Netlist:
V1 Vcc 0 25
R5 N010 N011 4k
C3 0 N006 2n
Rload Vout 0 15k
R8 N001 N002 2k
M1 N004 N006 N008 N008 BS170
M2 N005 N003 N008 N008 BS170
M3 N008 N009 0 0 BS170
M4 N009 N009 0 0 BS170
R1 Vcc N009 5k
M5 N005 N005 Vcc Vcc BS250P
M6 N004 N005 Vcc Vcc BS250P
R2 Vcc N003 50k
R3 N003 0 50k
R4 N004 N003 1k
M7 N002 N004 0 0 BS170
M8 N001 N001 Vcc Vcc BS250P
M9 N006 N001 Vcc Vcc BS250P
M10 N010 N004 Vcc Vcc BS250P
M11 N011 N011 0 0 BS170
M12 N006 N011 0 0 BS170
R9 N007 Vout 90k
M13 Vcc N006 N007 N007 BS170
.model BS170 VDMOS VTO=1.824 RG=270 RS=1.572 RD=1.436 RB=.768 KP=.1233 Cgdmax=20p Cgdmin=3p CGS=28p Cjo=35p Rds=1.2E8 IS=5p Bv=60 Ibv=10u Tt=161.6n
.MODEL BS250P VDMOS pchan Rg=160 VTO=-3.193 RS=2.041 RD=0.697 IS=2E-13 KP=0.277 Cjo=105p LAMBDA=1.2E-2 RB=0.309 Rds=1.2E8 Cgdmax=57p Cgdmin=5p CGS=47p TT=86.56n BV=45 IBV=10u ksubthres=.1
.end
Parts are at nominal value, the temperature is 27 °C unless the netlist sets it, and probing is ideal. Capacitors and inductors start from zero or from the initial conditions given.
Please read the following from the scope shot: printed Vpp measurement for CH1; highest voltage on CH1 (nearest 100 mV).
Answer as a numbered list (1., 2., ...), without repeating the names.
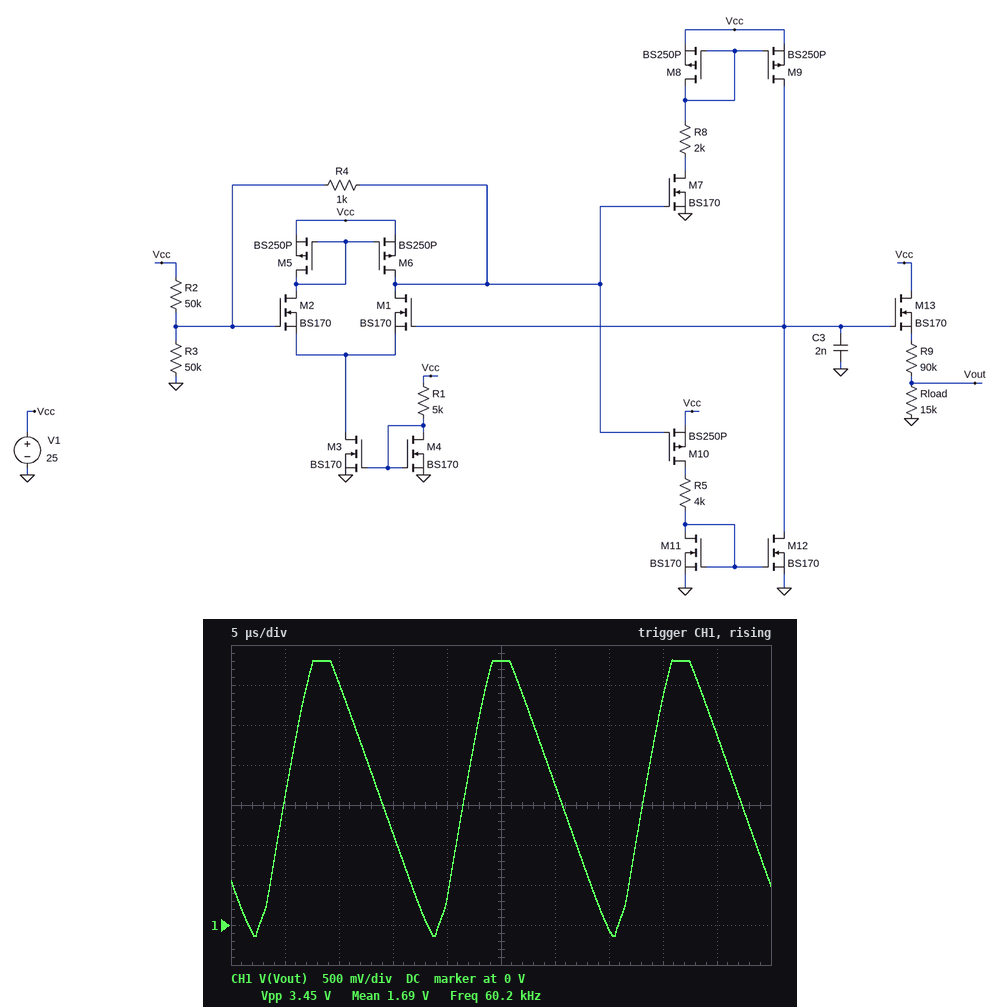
1. 3.45 V
2. 3.3 V
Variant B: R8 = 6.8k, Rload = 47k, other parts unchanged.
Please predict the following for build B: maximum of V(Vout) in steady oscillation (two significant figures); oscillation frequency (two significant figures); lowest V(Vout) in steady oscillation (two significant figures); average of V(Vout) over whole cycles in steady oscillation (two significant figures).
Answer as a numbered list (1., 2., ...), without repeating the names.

1. 7.7 V
2. 38 kHz
3. -330 mV
4. 3.7 V
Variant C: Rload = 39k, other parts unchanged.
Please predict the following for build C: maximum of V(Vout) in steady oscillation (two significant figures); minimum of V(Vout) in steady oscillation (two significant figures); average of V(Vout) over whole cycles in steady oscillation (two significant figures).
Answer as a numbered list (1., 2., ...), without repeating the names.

1. 7.0 V
2. -300 mV
3. 3.6 V
